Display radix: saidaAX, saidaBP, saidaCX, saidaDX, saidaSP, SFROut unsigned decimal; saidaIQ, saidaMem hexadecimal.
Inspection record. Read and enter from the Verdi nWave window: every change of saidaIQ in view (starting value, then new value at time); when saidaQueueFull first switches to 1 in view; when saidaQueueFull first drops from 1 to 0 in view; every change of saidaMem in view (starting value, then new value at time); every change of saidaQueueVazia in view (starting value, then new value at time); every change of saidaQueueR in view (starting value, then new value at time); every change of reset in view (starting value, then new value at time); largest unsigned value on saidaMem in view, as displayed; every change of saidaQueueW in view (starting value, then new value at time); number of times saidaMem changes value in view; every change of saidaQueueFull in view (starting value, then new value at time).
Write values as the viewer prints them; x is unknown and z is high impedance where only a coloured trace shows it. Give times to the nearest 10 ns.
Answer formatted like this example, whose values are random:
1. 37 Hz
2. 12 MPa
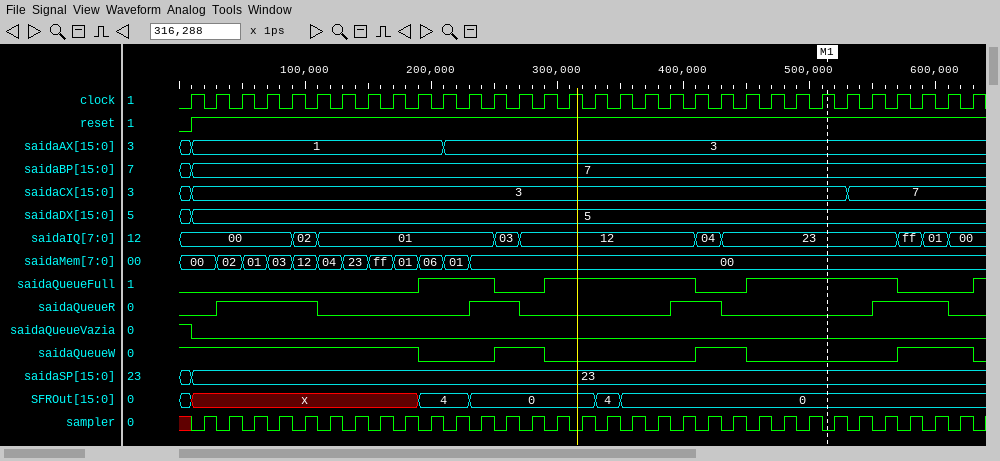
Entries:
1. 00, 02 at 90 ns, 01 at 110 ns, 03 at 250 ns, 12 at 270 ns, 04 at 410 ns, 23 at 430 ns, ff at 570 ns, 01 at 590 ns, 00 at 610 ns
2. 190 ns
3. 250 ns
4. 00, 02 at 30 ns, 01 at 50 ns, 03 at 70 ns, 12 at 90 ns, 04 at 110 ns, 23 at 130 ns, ff at 150 ns, 01 at 170 ns, 06 at 190 ns, 01 at 210 ns, 00 at 230 ns
5. 1, 0 at 10 ns
6. 0, 1 at 30 ns, 0 at 110 ns, 1 at 230 ns, 0 at 270 ns, 1 at 390 ns, 0 at 430 ns, 1 at 550 ns, 0 at 610 ns
7. 0, 1 at 10 ns
8. ff
9. 1, 0 at 190 ns, 1 at 250 ns, 0 at 290 ns, 1 at 410 ns, 0 at 450 ns, 1 at 570 ns, 0 at 630 ns
10. 11
11. 0, 1 at 190 ns, 0 at 250 ns, 1 at 290 ns, 0 at 410 ns, 1 at 450 ns, 0 at 570 ns, 1 at 630 ns
